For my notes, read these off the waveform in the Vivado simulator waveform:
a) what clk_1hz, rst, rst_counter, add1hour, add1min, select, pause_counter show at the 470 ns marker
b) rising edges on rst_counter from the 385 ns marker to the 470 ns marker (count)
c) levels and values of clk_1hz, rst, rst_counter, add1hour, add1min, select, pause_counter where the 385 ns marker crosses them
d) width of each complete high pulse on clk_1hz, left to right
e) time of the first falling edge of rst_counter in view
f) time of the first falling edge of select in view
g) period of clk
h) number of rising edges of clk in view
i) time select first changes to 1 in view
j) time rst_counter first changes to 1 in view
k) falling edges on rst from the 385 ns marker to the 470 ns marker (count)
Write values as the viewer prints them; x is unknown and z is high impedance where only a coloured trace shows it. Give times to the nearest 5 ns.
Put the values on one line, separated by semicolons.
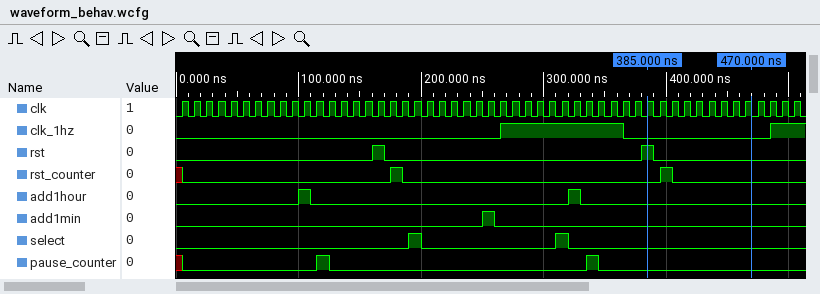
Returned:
clk_1hz=0, rst=0, rst_counter=0, add1hour=0, add1min=0, select=0, pause_counter=0; 1; clk_1hz=0, rst=1, rst_counter=0, add1hour=0, add1min=0, select=0, pause_counter=0; 100 ns; 185 ns; 200 ns; 10 ns; 51; 190 ns; 175 ns; 1
